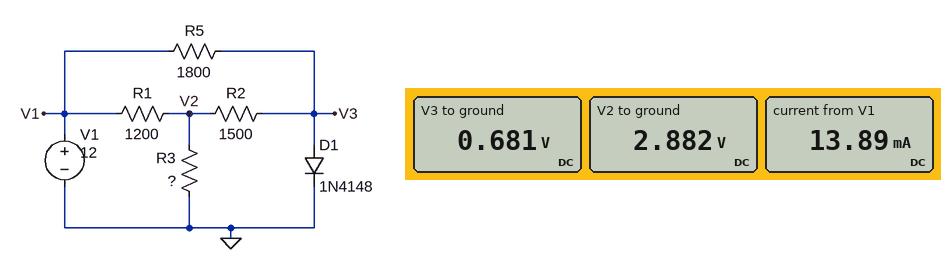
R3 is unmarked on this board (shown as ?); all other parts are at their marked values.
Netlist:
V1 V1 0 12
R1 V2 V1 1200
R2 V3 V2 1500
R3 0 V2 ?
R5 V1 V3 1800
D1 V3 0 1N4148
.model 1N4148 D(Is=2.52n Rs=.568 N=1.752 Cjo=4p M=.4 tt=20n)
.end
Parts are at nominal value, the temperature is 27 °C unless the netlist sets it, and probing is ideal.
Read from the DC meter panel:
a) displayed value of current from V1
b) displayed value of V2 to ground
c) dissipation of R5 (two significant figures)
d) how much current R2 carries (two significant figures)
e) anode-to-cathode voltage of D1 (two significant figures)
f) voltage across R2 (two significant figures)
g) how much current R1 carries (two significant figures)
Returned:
13.89 mA
2.882 V
71 mW
1.5 mA
680 mV
2.2 V
7.6 mA
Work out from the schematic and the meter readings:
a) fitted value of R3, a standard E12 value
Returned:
470 Ω
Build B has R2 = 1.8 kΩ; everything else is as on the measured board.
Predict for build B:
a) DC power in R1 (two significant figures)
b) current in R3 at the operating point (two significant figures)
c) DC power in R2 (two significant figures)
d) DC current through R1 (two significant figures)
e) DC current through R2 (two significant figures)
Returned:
68 mW
6.3 mA
2.9 mW
7.5 mA
1.3 mA
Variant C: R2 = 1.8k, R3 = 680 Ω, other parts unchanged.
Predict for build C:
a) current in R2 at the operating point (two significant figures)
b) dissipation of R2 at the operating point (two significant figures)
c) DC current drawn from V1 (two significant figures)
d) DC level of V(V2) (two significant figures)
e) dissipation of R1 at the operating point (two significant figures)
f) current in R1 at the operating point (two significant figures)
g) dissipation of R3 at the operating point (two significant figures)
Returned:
1.6 mA
4.8 mW
13 mA
3.6 V
58 mW
7.0 mA
19 mW
